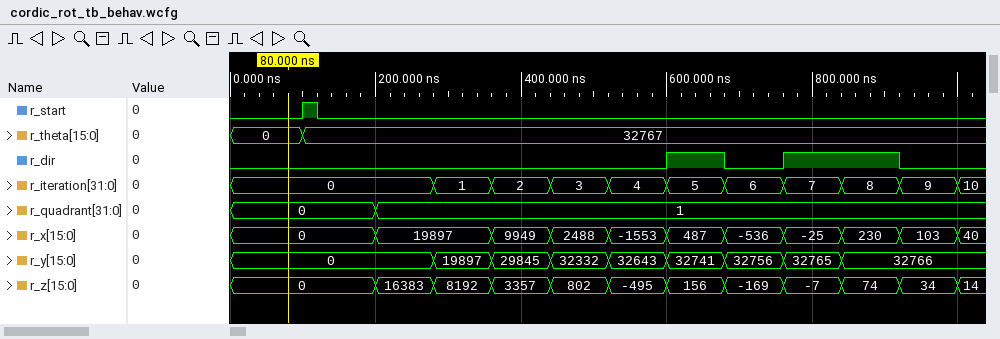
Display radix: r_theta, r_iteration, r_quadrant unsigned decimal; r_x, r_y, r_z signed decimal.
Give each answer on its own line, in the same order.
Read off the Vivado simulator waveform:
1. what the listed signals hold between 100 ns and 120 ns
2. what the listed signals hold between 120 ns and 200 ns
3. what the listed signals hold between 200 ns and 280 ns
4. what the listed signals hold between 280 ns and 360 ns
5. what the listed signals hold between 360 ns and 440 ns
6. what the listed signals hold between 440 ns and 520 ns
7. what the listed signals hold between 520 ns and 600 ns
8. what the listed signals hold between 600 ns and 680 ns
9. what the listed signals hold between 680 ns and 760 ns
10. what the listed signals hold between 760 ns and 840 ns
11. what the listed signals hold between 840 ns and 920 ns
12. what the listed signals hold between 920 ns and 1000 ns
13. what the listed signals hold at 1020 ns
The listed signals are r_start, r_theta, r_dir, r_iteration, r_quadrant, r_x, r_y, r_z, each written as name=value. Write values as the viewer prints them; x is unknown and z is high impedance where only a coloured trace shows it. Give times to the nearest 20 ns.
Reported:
r_start=1, r_theta=32767, r_dir=0, r_iteration=0, r_quadrant=0, r_x=0, r_y=0, r_z=0
r_start=0, r_theta=32767, r_dir=0, r_iteration=0, r_quadrant=0, r_x=0, r_y=0, r_z=0
r_start=0, r_theta=32767, r_dir=0, r_iteration=0, r_quadrant=1, r_x=19897, r_y=0, r_z=16383
r_start=0, r_theta=32767, r_dir=0, r_iteration=1, r_quadrant=1, r_x=19897, r_y=19897, r_z=8192
r_start=0, r_theta=32767, r_dir=0, r_iteration=2, r_quadrant=1, r_x=9949, r_y=29845, r_z=3357
r_start=0, r_theta=32767, r_dir=0, r_iteration=3, r_quadrant=1, r_x=2488, r_y=32332, r_z=802
r_start=0, r_theta=32767, r_dir=0, r_iteration=4, r_quadrant=1, r_x=-1553, r_y=32643, r_z=-495
r_start=0, r_theta=32767, r_dir=1, r_iteration=5, r_quadrant=1, r_x=487, r_y=32741, r_z=156
r_start=0, r_theta=32767, r_dir=0, r_iteration=6, r_quadrant=1, r_x=-536, r_y=32756, r_z=-169
r_start=0, r_theta=32767, r_dir=1, r_iteration=7, r_quadrant=1, r_x=-25, r_y=32765, r_z=-7
r_start=0, r_theta=32767, r_dir=1, r_iteration=8, r_quadrant=1, r_x=230, r_y=32766, r_z=74
r_start=0, r_theta=32767, r_dir=0, r_iteration=9, r_quadrant=1, r_x=103, r_y=32766, r_z=34
r_start=0, r_theta=32767, r_dir=0, r_iteration=10, r_quadrant=1, r_x=40, r_y=32766, r_z=14
